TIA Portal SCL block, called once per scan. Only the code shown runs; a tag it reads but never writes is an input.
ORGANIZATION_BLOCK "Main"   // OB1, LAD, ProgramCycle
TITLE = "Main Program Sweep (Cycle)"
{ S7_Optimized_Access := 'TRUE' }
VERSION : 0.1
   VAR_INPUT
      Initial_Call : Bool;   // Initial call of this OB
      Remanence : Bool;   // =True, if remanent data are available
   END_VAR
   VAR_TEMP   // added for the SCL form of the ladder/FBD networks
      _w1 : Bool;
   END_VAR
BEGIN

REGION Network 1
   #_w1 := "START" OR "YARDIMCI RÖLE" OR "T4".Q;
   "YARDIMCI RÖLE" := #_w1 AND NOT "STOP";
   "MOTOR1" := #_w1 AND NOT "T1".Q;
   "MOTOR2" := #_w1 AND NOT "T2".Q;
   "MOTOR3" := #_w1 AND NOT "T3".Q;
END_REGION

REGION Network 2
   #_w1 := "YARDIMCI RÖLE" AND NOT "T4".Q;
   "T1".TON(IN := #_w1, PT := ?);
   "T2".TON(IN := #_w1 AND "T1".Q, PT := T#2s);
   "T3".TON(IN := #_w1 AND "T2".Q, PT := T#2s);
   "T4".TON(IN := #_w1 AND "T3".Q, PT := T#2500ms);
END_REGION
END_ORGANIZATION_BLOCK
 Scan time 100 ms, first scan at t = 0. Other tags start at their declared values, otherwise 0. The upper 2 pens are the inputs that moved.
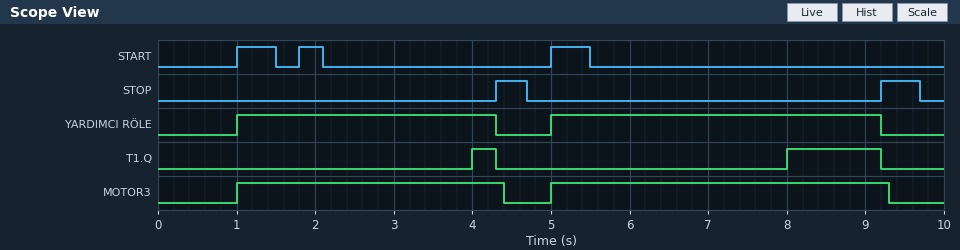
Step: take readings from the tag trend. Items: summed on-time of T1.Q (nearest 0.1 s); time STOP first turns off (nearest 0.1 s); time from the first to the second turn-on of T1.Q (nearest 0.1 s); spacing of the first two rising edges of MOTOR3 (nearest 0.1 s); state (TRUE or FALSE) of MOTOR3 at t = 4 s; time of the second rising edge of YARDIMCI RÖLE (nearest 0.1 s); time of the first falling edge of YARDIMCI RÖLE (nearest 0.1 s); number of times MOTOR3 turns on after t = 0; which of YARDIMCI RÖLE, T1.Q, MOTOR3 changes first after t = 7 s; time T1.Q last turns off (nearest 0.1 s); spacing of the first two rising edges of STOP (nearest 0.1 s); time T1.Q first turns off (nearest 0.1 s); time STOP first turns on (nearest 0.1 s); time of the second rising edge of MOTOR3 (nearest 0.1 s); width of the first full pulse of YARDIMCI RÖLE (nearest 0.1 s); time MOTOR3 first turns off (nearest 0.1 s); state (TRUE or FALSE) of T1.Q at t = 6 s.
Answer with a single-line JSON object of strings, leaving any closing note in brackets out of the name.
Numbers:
{"summed on-time of T1.Q": "1.5 s", "time STOP first turns off": "4.7 s", "time from the first to the second turn-on of T1.Q": "4.0 s", "spacing of the first two rising edges of MOTOR3": "4.0 s", "state (TRUE or FALSE) of MOTOR3 at t = 4 s": "TRUE", "time of the second rising edge of YARDIMCI RÖLE": "5.0 s", "time of the first falling edge of YARDIMCI RÖLE": "4.3 s", "number of times MOTOR3 turns on after t = 0": "2", "which of YARDIMCI RÖLE, T1.Q, MOTOR3 changes first after t = 7 s": "T1.Q", "time T1.Q last turns off": "9.2 s", "spacing of the first two rising edges of STOP": "4.9 s", "time T1.Q first turns off": "4.3 s", "time STOP first turns on": "4.3 s", "time of the second rising edge of MOTOR3": "5.0 s", "width of the first full pulse of YARDIMCI RÖLE": "3.3 s", "time MOTOR3 first turns off": "4.4 s", "state (TRUE or FALSE) of T1.Q at t = 6 s": "FALSE"}
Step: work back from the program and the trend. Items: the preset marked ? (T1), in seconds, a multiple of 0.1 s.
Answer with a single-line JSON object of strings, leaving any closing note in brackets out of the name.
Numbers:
{"the preset marked ? (T1), in seconds, a multiple of 0.1 s": "3.0 s"}
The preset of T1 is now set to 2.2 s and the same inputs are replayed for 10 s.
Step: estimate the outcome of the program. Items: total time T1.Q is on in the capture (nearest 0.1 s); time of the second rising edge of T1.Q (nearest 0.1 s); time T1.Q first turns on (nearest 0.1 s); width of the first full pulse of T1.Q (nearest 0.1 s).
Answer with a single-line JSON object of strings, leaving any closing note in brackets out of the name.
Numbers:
{"total time T1.Q is on in the capture": "3.1 s", "time of the second rising edge of T1.Q": "7.2 s", "time T1.Q first turns on": "3.2 s", "width of the first full pulse of T1.Q": "1.1 s"}
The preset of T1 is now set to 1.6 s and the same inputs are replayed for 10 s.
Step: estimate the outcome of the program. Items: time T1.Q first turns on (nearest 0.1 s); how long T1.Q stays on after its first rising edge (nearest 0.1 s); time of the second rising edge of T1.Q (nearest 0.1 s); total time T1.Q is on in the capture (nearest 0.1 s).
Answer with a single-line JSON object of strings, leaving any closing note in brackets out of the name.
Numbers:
{"time T1.Q first turns on": "2.6 s", "how long T1.Q stays on after its first rising edge": "1.7 s", "time of the second rising edge of T1.Q": "6.6 s", "total time T1.Q is on in the capture": "4.3 s"}
